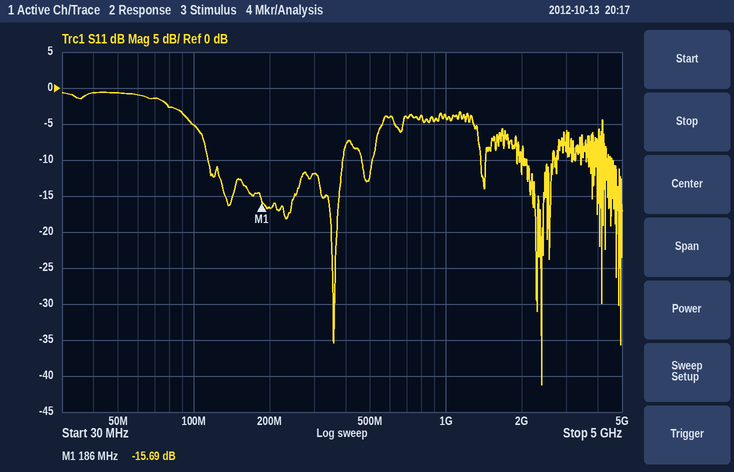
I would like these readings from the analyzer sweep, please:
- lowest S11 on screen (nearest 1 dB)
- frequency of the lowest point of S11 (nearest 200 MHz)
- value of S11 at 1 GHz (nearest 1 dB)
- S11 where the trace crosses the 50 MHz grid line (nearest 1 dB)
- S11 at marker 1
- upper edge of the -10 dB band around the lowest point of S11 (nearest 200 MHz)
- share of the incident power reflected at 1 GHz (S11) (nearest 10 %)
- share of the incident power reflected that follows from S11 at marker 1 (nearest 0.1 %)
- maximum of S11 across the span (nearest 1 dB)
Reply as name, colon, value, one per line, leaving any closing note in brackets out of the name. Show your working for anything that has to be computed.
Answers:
lowest S11 on screen: -41 dB
frequency of the lowest point of S11: 2.4 GHz
value of S11 at 1 GHz: -4 dB
S11 where the trace crosses the 50 MHz grid line: -1 dB
S11 at marker 1: -15.69 dB
upper edge of the -10 dB band around the lowest point of S11: 2.6 GHz
share of the incident power reflected at 1 GHz (S11): 10^(-4/10) ≈ 40 %
share of the incident power reflected that follows from S11 at marker 1: 10^(-15.69/10) ≈ 2.7 %
maximum of S11 across the span: -1 dB
